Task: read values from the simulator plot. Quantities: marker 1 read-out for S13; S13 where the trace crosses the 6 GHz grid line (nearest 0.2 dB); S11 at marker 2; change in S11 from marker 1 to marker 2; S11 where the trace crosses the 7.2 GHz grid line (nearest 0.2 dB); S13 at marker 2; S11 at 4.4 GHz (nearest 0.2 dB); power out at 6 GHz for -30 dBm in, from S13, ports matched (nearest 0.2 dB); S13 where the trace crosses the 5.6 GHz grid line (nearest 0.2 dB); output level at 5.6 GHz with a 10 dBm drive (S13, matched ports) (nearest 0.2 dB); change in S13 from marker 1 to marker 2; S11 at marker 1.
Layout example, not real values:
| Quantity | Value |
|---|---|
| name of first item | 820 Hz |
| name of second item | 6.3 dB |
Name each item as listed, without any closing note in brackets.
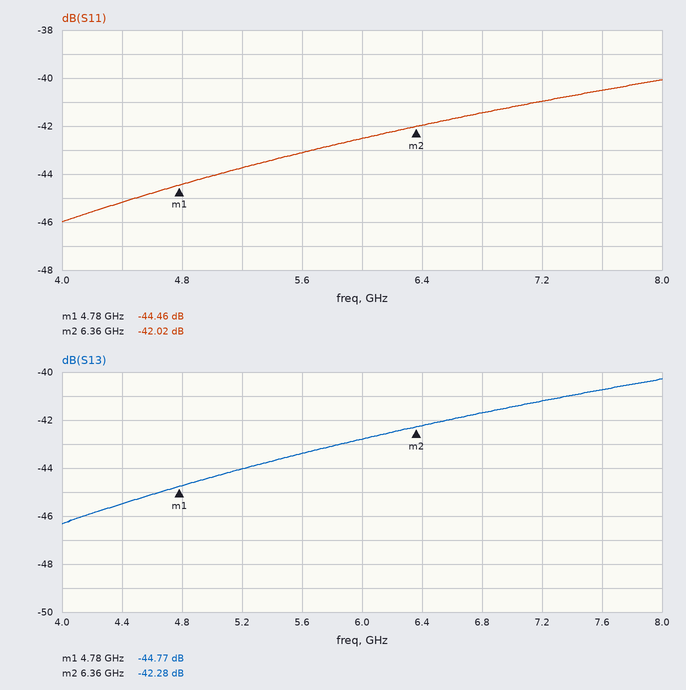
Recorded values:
| Quantity | Value |
|---|---|
| marker 1 read-out for S13 | -44.77 dB |
| S13 where the trace crosses the 6 GHz grid line | -42.8 dB |
| S11 at marker 2 | -42.02 dB |
| change in S11 from marker 1 to marker 2 | 2.44 dB |
| S11 where the trace crosses the 7.2 GHz grid line | -41.0 dB |
| S13 at marker 2 | -42.28 dB |
| S11 at 4.4 GHz | -45.2 dB |
| power out at 6 GHz for -30 dBm in, from S13, ports matched | -72.8 dBm |
| S13 where the trace crosses the 5.6 GHz grid line | -43.4 dB |
| output level at 5.6 GHz with a 10 dBm drive (S13, matched ports) | -33.4 dBm |
| change in S13 from marker 1 to marker 2 | 2.49 dB |
| S11 at marker 1 | -44.46 dB |
